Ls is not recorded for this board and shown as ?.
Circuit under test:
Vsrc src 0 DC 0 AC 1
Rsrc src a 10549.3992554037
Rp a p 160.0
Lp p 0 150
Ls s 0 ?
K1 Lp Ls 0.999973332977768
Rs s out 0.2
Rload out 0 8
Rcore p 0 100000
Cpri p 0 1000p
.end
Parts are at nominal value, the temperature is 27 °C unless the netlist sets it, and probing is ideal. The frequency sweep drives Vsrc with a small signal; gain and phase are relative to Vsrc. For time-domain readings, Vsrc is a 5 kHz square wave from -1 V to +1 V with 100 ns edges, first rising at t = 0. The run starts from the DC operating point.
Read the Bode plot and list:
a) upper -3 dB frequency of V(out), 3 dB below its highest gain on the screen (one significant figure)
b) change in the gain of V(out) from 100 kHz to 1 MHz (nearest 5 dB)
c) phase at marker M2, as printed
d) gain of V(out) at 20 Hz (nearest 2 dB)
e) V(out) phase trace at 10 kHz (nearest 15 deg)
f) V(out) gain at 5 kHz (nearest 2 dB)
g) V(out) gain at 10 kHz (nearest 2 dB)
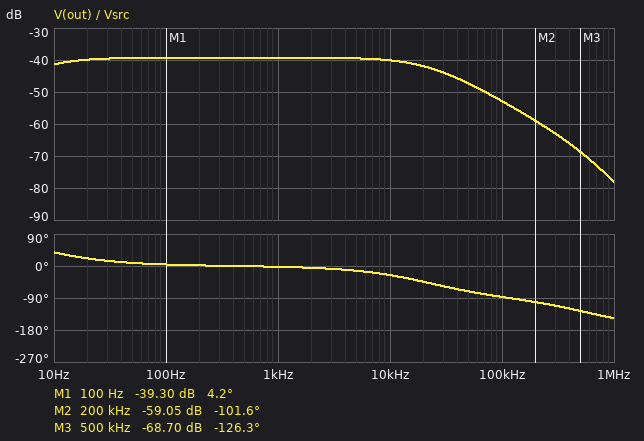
20 kHz
-25 dB
-101.6 deg
-40 dB
-30 deg
-40 dB
-40 dB
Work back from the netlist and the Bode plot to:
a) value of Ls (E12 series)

39 mH
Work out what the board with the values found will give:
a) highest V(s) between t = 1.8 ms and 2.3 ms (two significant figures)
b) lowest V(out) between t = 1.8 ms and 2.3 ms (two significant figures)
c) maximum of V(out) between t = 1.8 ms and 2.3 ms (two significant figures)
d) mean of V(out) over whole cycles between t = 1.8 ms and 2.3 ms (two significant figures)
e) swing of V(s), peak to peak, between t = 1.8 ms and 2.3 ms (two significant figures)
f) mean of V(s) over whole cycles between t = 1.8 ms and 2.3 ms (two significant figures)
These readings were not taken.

21 mV
-1.1 mV
21 mV
9.8 mV
22 mV
10 mV
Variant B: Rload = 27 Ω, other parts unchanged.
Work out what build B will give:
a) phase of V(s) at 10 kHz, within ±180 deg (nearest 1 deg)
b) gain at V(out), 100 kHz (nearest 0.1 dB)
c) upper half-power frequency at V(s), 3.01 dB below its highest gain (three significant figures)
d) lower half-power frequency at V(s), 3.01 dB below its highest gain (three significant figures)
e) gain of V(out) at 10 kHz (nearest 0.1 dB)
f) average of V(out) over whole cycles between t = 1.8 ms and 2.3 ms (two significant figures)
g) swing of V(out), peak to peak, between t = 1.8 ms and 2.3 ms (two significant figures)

-29 deg
-52.6 dB
18.0 kHz
9.39 Hz
-38.7 dB
12 mV
27 mV
